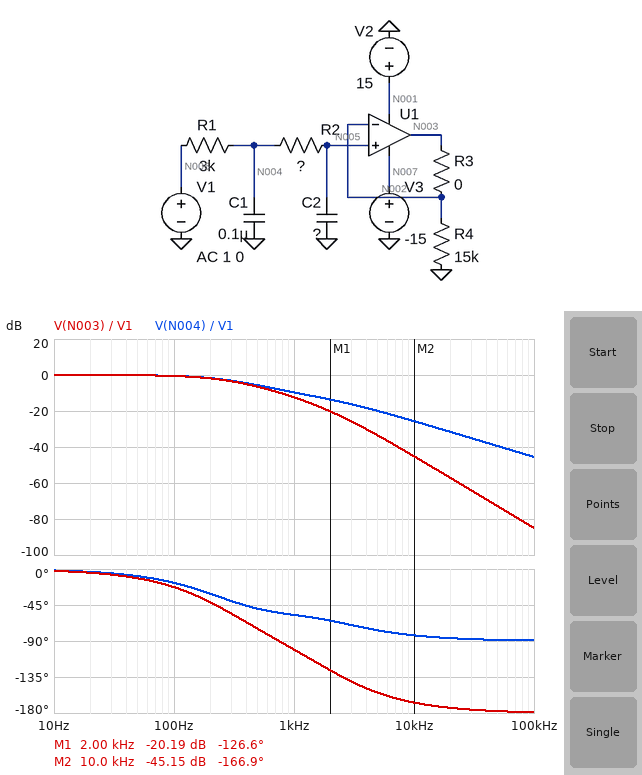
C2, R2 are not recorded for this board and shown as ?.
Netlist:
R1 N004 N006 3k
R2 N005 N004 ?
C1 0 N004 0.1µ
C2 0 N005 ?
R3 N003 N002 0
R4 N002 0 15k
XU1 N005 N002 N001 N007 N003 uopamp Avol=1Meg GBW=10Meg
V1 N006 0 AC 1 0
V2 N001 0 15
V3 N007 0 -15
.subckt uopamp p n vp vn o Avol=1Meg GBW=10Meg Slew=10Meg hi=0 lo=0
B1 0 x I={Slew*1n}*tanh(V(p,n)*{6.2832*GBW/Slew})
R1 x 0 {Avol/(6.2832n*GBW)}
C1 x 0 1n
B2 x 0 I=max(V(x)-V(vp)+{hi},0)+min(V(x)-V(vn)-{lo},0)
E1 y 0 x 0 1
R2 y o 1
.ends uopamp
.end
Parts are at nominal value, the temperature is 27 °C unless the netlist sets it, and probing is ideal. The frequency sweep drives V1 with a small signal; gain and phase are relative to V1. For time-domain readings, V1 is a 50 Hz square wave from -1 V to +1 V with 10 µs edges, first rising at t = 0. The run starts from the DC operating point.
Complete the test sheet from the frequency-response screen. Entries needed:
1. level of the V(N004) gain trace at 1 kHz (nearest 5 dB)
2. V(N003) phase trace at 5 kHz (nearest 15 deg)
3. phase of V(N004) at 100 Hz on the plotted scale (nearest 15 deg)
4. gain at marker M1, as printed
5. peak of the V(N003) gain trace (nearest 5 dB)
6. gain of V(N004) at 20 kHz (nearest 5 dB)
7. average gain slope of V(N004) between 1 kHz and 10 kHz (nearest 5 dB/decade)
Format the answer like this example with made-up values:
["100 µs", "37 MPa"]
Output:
["-10 dB", "-150 deg", "-15 deg", "-20.19 dB", "0 dB", "-30 dB", "-15 dB/decade"]
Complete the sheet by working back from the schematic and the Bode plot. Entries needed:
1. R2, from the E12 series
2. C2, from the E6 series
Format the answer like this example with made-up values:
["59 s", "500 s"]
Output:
["2.2 kΩ", "68 nF"]
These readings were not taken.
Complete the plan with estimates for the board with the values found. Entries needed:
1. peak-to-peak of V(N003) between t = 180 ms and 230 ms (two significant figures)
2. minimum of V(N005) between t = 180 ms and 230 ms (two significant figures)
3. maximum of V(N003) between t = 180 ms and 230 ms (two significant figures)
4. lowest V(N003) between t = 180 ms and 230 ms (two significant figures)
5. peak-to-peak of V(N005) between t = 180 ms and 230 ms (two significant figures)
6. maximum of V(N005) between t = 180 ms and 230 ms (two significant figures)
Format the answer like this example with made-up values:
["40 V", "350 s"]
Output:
["2.0 V", "-1.0 V", "1.0 V", "-1.0 V", "2.0 V", "1.0 V"]
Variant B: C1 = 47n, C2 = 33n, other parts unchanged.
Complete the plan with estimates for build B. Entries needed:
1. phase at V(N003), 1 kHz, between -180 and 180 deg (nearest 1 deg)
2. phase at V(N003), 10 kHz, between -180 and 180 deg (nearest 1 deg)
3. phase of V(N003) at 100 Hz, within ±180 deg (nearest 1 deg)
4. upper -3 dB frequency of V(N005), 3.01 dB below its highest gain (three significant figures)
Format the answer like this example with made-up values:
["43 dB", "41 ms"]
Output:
["-73 deg", "-154 deg", "-11 deg", "568 Hz"]
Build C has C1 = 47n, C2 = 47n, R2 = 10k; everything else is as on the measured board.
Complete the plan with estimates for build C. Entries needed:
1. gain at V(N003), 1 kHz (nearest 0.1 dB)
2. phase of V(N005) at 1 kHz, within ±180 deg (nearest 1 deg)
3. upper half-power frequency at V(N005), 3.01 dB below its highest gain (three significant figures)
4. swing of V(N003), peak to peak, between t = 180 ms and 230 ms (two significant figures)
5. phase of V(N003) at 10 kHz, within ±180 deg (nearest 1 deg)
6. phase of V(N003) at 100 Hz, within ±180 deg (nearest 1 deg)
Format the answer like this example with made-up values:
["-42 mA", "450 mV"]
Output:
["-14.0 dB", "-109 deg", "239 Hz", "2.0 V", "-170 deg", "-26 deg"]
